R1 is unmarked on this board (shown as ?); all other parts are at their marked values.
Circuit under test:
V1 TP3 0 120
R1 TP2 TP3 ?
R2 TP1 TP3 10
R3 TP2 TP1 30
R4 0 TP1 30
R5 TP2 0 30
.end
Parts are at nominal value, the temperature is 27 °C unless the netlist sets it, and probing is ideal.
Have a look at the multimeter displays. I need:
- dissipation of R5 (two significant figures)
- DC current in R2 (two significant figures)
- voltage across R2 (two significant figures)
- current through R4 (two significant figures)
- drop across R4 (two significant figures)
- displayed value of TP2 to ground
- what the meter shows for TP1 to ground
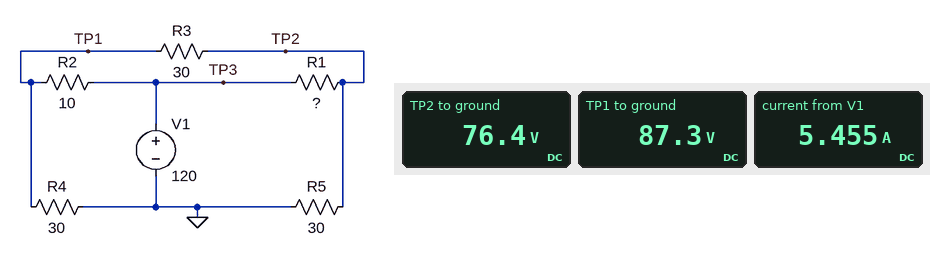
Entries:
190 W
3.3 A
33 V
2.9 A
87 V
76.4 V
87.3 V
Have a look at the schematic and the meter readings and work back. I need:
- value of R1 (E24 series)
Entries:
20 Ω
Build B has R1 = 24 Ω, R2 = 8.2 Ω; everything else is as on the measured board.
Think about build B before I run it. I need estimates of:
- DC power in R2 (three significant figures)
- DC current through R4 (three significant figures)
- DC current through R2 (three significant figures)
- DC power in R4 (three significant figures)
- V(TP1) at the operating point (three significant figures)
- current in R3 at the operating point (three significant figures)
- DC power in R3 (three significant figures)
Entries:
105 W
3.02 A
3.58 A
274 W
90.7 V
554 mA
9.21 W
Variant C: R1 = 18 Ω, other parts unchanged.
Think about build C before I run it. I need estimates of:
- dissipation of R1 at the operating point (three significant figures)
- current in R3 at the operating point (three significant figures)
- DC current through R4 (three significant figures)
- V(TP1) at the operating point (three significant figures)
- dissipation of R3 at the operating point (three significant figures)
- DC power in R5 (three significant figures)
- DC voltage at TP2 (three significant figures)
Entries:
95.9 W
308 mA
2.92 A
87.7 V
2.84 W
205 W
78.5 V
